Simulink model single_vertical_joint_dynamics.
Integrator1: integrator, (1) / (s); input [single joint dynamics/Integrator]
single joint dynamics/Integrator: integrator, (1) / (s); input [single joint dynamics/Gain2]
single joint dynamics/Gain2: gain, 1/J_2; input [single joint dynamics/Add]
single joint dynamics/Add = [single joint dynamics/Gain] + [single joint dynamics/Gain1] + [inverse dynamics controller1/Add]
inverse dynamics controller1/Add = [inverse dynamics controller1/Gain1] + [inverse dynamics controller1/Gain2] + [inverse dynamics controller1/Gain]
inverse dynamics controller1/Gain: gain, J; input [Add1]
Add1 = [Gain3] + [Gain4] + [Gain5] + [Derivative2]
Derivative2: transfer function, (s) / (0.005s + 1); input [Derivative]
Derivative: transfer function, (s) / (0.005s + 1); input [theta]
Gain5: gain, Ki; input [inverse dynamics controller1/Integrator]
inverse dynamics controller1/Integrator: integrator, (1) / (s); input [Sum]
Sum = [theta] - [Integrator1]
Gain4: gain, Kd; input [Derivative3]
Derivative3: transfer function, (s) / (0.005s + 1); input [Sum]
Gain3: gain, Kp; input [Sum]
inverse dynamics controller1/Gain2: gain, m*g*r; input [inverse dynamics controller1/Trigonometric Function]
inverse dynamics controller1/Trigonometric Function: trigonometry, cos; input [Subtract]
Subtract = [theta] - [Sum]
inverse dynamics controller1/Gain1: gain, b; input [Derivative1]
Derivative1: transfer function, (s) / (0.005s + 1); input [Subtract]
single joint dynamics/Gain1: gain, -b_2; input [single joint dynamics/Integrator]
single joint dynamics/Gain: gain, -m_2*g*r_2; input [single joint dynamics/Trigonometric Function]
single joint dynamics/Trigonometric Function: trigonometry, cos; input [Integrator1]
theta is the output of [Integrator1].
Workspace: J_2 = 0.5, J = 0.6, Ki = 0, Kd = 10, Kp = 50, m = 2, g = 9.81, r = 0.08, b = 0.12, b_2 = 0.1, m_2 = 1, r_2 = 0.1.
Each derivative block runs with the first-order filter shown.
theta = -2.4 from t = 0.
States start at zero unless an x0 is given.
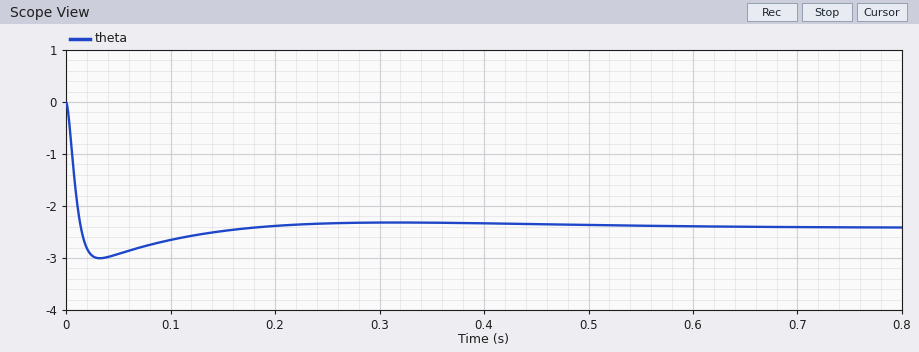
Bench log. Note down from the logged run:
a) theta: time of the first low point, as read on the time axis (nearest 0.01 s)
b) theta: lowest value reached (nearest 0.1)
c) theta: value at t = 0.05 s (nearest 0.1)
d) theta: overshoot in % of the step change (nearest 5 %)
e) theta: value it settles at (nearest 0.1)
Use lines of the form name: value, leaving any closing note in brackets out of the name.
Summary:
theta: time of the first low point, as read on the time axis: 0.03 s
theta: lowest value reached: -3.0
theta: value at t = 0.05 s: -2.9
theta: overshoot in % of the step change: 25 %
theta: value it settles at: -2.4
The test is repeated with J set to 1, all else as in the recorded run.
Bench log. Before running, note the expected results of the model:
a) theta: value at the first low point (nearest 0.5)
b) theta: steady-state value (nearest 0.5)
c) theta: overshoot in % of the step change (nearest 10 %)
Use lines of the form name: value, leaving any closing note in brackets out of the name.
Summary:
theta: value at the first low point: -4.5
theta: steady-state value: -2.5
theta: overshoot in % of the step change: 90 %
